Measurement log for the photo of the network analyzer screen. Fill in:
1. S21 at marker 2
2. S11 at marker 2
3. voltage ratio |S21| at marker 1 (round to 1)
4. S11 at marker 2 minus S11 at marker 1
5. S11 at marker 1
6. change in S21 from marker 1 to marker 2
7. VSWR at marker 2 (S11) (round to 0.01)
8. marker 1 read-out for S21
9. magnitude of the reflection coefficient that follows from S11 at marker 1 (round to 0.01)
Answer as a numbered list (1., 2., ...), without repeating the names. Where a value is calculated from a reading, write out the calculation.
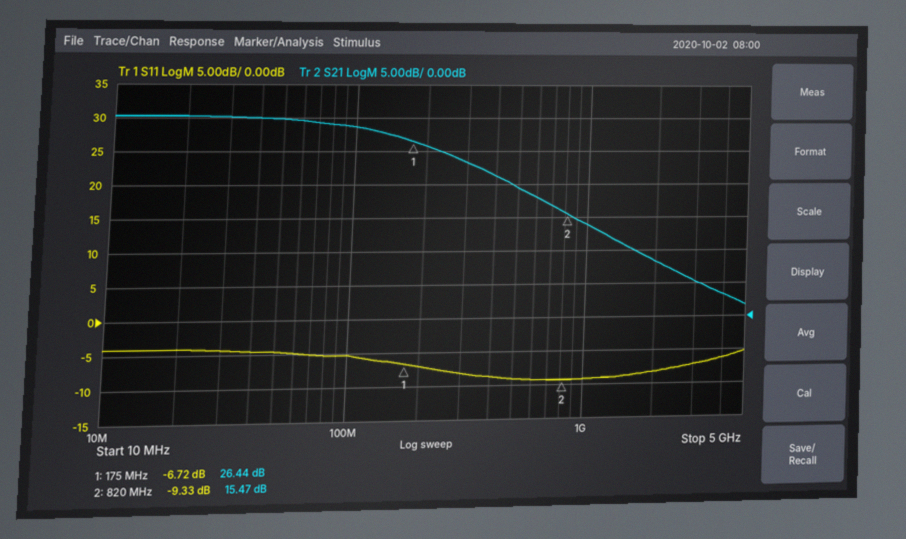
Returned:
1. 15.47 dB
2. -9.33 dB
3. 10^(26.44/20) ≈ 21
4. -9.33 − (-6.72) = -2.61 dB
5. -6.72 dB
6. 15.47 − (26.44) = -10.97 dB
7. (1 + 0.3416)/(1 − 0.3416) ≈ 2.04
8. 26.44 dB
9. 10^(-6.72/20) ≈ 0.46
